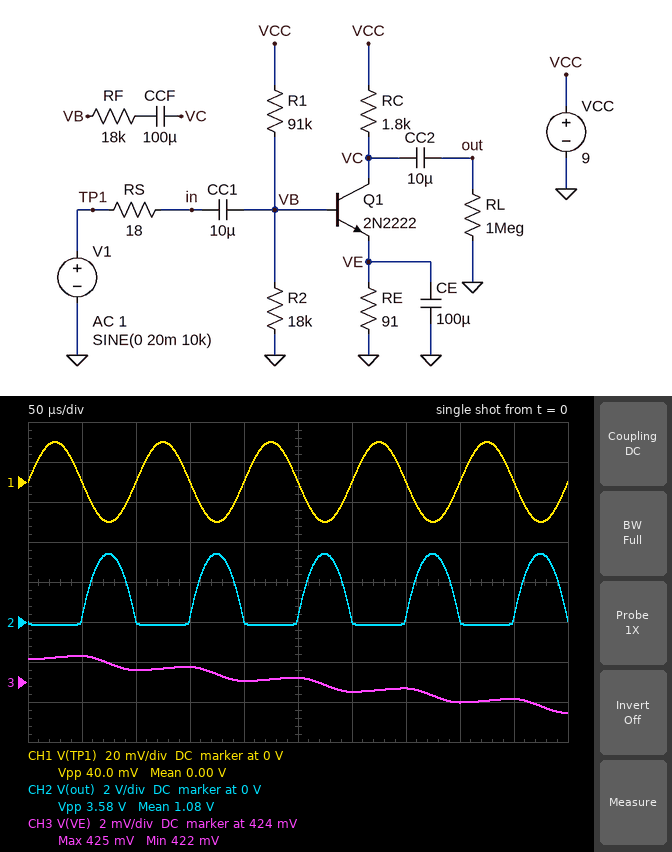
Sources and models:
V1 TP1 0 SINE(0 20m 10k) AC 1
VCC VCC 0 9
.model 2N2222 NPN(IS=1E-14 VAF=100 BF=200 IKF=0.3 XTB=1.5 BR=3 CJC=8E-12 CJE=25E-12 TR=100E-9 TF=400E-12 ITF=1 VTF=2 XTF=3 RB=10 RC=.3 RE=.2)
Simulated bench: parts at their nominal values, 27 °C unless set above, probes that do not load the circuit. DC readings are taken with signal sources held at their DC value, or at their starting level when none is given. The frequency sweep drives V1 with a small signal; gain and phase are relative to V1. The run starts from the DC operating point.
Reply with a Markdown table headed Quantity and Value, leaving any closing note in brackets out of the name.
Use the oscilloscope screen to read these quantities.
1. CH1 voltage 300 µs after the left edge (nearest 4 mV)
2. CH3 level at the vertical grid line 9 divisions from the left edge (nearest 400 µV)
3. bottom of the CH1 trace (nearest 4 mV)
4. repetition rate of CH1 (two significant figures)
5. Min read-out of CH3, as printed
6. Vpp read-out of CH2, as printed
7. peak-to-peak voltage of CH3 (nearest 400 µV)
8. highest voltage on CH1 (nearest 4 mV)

| Quantity | Value |
|---|---|
| CH1 voltage 300 µs after the left edge | 0 V |
| CH3 level at the vertical grid line 9 divisions from the left edge | 423.2 mV |
| bottom of the CH1 trace | -20 mV |
| repetition rate of CH1 | 10 kHz |
| Min read-out of CH3, as printed | 422 mV |
| Vpp read-out of CH2, as printed | 3.58 V |
| peak-to-peak voltage of CH3 | 2.8 mV |
| highest voltage on CH1 | 20 mV |
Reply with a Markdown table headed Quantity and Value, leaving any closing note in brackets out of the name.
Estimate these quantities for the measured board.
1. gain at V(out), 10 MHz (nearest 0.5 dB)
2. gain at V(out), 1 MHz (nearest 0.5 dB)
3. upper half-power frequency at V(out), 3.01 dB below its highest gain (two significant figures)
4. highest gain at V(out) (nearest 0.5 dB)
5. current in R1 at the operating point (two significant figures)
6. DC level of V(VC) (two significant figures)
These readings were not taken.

| Quantity | Value |
|---|---|
| gain at V(out), 10 MHz | 28.5 dB |
| gain at V(out), 1 MHz | 43.0 dB |
| upper half-power frequency at V(out), 3.01 dB below its highest gain | 1.6 MHz |
| highest gain at V(out) | 44.5 dB |
| current in R1 at the operating point | 87 µA |
| DC level of V(VC) | 630 mV |
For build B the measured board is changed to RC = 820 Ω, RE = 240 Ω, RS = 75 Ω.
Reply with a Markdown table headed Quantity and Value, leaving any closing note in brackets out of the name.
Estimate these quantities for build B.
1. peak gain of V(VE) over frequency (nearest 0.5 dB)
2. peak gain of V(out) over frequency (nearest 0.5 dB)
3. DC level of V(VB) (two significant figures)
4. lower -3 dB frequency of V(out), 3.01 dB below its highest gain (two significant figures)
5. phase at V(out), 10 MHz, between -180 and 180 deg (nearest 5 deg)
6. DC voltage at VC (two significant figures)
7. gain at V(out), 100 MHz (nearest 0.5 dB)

| Quantity | Value |
|---|---|
| peak gain of V(VE) over frequency | -4.0 dB |
| peak gain of V(out) over frequency | 35.0 dB |
| DC level of V(VB) | 1.3 V |
| lower -3 dB frequency of V(out), 3.01 dB below its highest gain | 170 Hz |
| phase at V(out), 10 MHz, between -180 and 180 deg | 120 deg |
| DC voltage at VC | 6.9 V |
| gain at V(out), 100 MHz | 10.0 dB |
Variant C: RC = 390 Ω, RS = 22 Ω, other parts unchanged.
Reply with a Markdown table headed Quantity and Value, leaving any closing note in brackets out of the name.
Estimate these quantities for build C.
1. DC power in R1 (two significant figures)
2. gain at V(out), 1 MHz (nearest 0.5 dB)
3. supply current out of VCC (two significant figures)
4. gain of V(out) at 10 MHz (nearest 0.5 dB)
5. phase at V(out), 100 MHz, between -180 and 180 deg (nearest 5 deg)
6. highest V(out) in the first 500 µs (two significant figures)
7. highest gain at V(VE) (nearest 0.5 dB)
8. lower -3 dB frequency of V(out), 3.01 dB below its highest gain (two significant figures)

| Quantity | Value |
|---|---|
| DC power in R1 | 680 µW |
| gain at V(out), 1 MHz | 35.5 dB |
| supply current out of VCC | 4.9 mA |
| gain of V(out) at 10 MHz | 33.5 dB |
| phase at V(out), 100 MHz, between -180 and 180 deg | 85 deg |
| highest V(out) in the first 500 µs | 970 mV |
| highest gain at V(VE) | -2.5 dB |
| lower -3 dB frequency of V(out), 3.01 dB below its highest gain | 330 Hz |
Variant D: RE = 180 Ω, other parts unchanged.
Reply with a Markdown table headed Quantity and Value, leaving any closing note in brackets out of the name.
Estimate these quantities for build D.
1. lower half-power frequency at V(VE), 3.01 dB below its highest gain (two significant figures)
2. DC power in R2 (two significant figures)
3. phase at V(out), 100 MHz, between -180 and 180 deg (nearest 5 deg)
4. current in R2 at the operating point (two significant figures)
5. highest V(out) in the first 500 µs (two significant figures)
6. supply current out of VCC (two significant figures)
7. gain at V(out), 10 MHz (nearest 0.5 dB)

| Quantity | Value |
|---|---|
| lower half-power frequency at V(VE), 3.01 dB below its highest gain | 5.1 Hz |
| DC power in R2 | 87 µW |
| phase at V(out), 100 MHz, between -180 and 180 deg | 75 deg |
| current in R2 at the operating point | 70 µA |
| highest V(out) in the first 500 µs | 2.5 V |
| supply current out of VCC | 3.2 mA |
| gain at V(out), 10 MHz | 37.0 dB |
